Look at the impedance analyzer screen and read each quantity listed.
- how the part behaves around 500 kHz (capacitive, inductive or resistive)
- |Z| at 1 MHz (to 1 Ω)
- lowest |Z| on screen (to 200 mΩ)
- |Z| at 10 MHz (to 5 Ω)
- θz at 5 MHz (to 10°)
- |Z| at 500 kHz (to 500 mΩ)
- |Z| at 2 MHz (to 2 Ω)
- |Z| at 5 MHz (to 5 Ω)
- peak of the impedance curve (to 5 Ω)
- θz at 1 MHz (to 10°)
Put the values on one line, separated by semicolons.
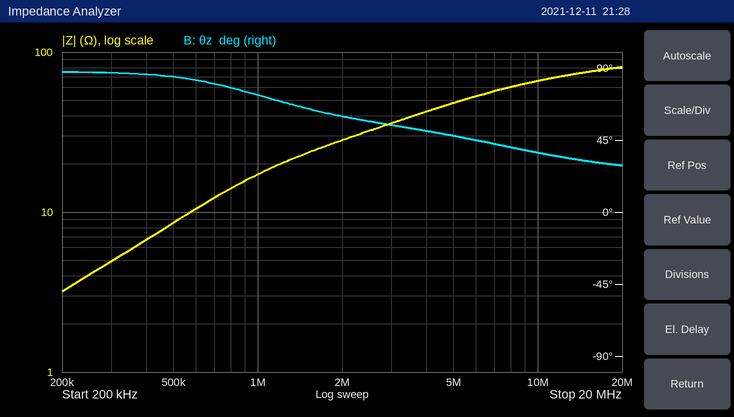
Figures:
inductive; 17 Ω; 3.2 Ω; 65 Ω; 50°; 8.5 Ω; 28 Ω; 50 Ω; 80 Ω; 70°
